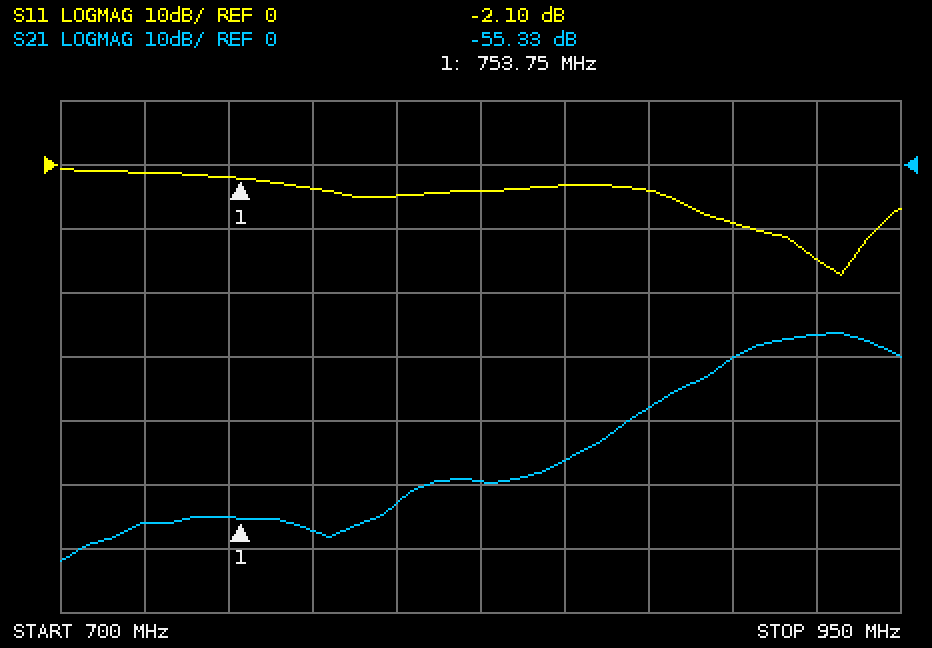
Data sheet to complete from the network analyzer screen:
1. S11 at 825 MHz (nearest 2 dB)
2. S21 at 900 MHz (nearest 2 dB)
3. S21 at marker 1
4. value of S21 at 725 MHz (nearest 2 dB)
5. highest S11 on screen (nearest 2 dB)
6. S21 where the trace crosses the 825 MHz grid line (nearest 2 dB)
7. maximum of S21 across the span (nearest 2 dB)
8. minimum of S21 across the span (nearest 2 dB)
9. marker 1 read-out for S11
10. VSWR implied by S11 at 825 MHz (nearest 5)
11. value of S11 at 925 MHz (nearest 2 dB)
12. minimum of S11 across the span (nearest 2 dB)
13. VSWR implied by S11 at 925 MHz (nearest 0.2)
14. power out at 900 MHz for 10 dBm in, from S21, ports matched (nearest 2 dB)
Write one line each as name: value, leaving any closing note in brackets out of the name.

S11 at 825 MHz: -4 dB
S21 at 900 MHz: -30 dB
S21 at marker 1: -55.33 dB
value of S21 at 725 MHz: -56 dB
highest S11 on screen: 0 dB
S21 where the trace crosses the 825 MHz grid line: -50 dB
maximum of S21 across the span: -26 dB
minimum of S21 across the span: -62 dB
marker 1 read-out for S11: -2.10 dB
VSWR implied by S11 at 825 MHz: 5
value of S11 at 925 MHz: -14 dB
minimum of S11 across the span: -18 dB
VSWR implied by S11 at 925 MHz: 1.4
power out at 900 MHz for 10 dBm in, from S21, ports matched: -20 dBm
